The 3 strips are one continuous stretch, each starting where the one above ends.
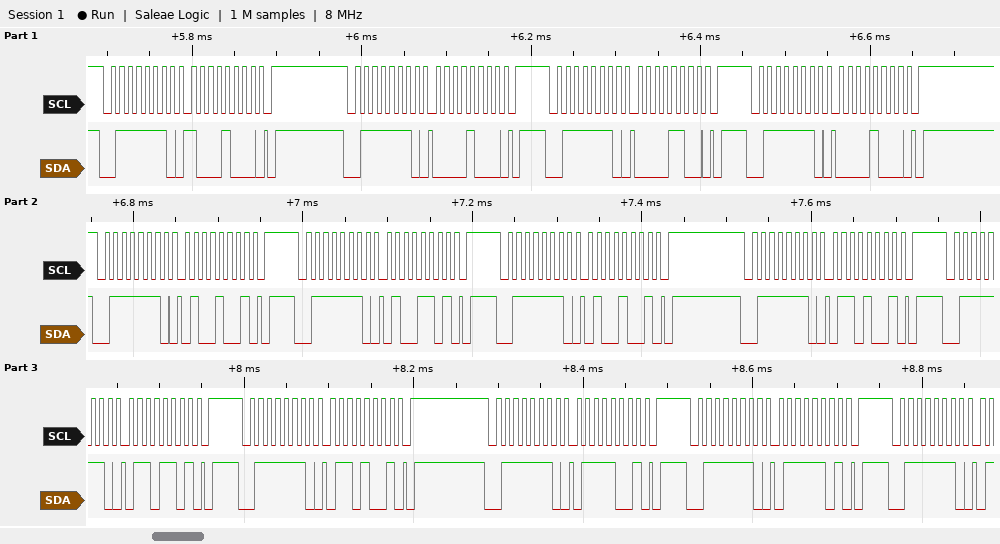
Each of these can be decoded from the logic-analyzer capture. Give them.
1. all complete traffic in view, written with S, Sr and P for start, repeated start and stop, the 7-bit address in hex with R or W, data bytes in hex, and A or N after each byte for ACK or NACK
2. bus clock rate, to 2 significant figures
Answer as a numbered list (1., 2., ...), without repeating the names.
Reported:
1. S 3FW A 88 A P S 3FW A 08 A P S 3FW A 0C A P S 3FW A 08 A P S 3FW A 49 A P S 3FW A 4D A P S 3FW A 49 A P S 3FW A 69 A P S 3FW A 6D A P S 3FW A 69 A P S 3FW A 79 A P S 3FW A 7D A P S 3FW A
2. 100 kHz
